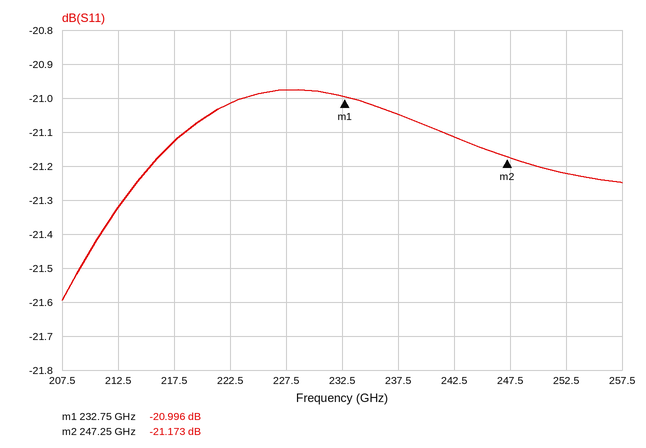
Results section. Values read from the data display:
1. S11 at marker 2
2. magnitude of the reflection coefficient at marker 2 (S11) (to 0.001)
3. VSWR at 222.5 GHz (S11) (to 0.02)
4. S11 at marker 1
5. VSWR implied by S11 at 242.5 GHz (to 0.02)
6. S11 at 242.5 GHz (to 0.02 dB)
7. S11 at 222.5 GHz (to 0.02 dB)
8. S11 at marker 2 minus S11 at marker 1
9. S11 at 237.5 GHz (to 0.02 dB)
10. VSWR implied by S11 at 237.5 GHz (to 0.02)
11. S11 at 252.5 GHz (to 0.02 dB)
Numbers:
-21.173 dB
0.087
1.20
-20.996 dB
1.20
-21.12 dB
-21.02 dB
-0.177 dB
-21.04 dB
1.20
-21.22 dB
